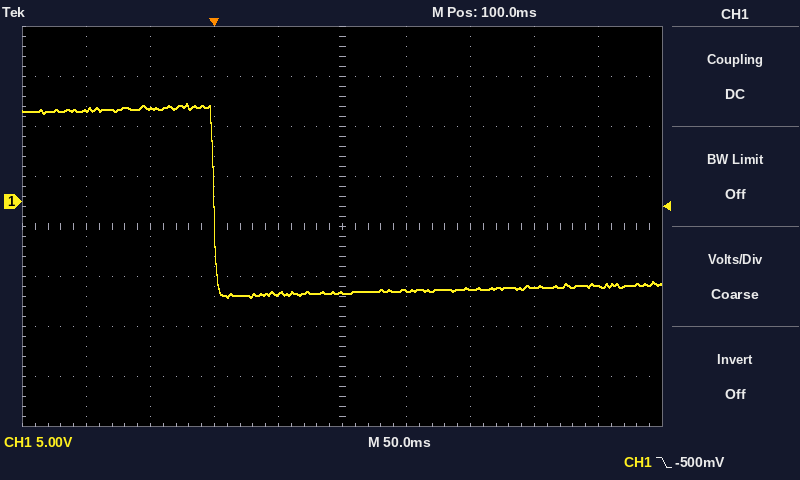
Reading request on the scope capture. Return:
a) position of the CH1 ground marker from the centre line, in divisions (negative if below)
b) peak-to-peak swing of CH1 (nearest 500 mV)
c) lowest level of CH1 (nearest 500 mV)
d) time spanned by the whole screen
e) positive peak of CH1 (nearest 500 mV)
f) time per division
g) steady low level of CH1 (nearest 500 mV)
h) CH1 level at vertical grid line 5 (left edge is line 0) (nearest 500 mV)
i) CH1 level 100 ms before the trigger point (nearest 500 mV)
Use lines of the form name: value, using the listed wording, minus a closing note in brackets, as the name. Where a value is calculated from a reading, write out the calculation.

position of the CH1 ground marker from the centre line, in divisions: +0.5 div
peak-to-peak swing of CH1: 10.0 V − (-9.5 V) = 19.5 V
lowest level of CH1: -9.5 V
time spanned by the whole screen: 500 ms
positive peak of CH1: 10.0 V
time per division: 50 ms
steady low level of CH1: -9.0 V
CH1 level at vertical grid line 5 (left edge is line 0): -9.0 V
CH1 level 100 ms before the trigger point: 9.0 V
